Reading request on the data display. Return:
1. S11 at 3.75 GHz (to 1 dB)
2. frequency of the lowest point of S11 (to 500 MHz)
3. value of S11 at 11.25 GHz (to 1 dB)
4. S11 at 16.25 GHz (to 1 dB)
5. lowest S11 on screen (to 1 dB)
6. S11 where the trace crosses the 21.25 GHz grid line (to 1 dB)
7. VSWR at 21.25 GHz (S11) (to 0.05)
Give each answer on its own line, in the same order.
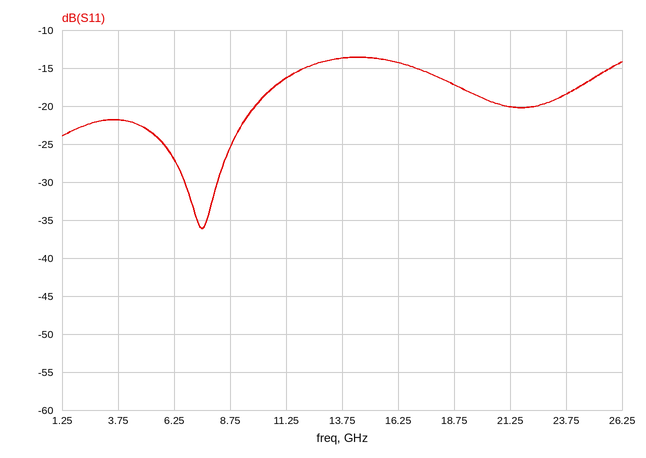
-22 dB
7.5 GHz
-16 dB
-14 dB
-36 dB
-20 dB
1.20
